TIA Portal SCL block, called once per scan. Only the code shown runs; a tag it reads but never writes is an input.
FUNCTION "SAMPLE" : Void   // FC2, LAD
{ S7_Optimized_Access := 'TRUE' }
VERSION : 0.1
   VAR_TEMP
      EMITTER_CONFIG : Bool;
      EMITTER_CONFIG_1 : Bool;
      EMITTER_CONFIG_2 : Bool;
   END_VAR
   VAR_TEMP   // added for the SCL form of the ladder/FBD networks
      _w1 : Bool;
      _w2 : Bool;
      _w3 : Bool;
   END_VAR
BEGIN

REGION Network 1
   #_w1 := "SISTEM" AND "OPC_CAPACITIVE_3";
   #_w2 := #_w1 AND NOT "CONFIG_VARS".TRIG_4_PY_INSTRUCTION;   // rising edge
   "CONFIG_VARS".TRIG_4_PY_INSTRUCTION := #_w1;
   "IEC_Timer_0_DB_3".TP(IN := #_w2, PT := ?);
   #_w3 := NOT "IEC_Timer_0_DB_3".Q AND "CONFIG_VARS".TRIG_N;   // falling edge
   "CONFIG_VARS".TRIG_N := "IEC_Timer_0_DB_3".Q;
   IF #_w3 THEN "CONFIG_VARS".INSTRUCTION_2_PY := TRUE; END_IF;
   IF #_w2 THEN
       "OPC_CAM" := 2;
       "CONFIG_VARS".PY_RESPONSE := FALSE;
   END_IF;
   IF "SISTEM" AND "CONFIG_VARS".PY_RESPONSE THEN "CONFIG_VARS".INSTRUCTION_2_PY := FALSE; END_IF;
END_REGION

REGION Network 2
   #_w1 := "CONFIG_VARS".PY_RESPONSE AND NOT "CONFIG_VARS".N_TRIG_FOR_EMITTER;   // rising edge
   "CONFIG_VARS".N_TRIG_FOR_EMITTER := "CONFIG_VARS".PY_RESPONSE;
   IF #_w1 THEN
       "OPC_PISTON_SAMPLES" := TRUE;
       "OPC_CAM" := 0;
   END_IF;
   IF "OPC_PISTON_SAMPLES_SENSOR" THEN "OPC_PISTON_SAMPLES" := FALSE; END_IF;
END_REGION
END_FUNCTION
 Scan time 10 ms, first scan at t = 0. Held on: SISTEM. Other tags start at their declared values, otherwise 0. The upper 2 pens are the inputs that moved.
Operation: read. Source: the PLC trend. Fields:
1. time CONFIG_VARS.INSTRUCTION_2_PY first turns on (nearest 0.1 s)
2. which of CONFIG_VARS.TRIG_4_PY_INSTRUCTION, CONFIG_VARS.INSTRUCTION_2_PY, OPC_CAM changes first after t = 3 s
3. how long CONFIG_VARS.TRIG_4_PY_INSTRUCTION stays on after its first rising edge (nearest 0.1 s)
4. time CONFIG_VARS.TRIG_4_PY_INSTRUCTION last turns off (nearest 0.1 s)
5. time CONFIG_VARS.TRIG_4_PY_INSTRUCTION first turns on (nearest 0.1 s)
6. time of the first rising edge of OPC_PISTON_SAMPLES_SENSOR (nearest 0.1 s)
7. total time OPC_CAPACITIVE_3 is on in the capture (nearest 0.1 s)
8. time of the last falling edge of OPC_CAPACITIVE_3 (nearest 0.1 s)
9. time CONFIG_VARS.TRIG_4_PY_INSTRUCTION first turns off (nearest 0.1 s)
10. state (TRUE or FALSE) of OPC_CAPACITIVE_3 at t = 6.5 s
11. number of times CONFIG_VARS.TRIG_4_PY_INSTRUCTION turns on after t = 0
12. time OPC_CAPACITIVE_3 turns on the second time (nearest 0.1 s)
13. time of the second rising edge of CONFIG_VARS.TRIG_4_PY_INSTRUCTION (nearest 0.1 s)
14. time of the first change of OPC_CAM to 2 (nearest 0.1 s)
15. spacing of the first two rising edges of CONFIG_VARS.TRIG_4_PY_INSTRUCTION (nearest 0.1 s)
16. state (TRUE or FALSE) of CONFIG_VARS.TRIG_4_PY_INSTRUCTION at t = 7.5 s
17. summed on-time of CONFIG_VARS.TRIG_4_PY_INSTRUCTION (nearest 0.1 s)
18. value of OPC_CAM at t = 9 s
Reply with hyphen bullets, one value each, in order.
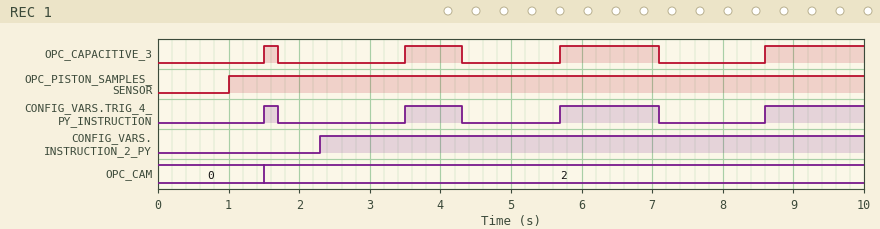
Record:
- 2.3 s
- CONFIG_VARS.TRIG_4_PY_INSTRUCTION
- 0.2 s
- 7.1 s
- 1.5 s
- 1.0 s
- 3.8 s
- 7.1 s
- 1.7 s
- TRUE
- 4
- 3.5 s
- 3.5 s
- 1.5 s
- 2.0 s
- FALSE
- 3.8 s
- 2
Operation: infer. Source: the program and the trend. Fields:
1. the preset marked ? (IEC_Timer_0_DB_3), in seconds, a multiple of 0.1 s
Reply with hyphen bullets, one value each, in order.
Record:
- 0.8 s
